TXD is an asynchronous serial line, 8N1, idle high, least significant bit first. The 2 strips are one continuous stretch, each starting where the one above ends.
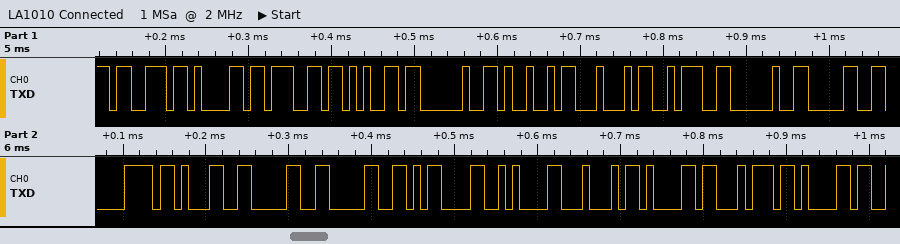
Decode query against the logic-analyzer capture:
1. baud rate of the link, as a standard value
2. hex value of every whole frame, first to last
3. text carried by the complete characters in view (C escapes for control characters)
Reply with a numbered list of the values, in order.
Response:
1. 115200 baud
2. 73 61 67 65 20 49 44 3A 20 30 78 31 30 30 0D 0A 44 61 74 61
3. "sage ID: 0x100\r\nData"
